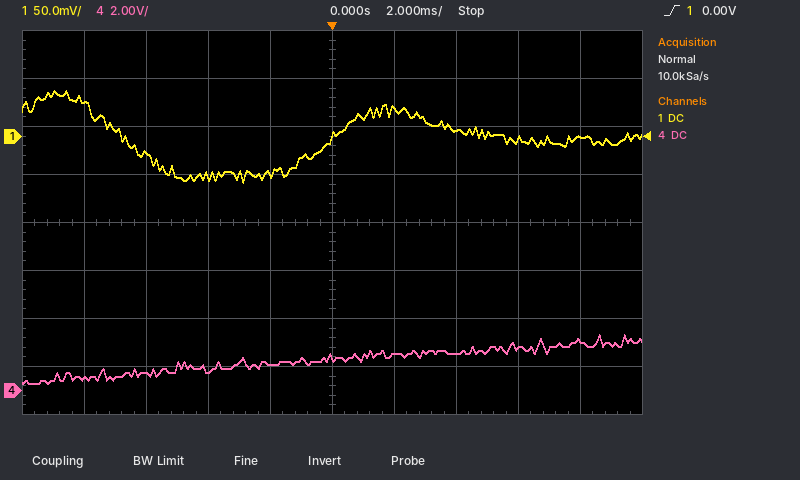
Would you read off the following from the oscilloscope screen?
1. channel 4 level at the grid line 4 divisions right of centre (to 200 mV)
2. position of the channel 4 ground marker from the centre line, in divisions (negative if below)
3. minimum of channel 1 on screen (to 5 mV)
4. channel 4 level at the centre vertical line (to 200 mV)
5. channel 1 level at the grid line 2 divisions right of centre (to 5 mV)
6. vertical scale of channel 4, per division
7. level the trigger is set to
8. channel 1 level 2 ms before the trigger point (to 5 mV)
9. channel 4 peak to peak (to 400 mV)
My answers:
2.0 V
-3.5 div
-50 mV
1.4 V
5 mV
2 V
0.00 V
-40 mV
2.0 V
